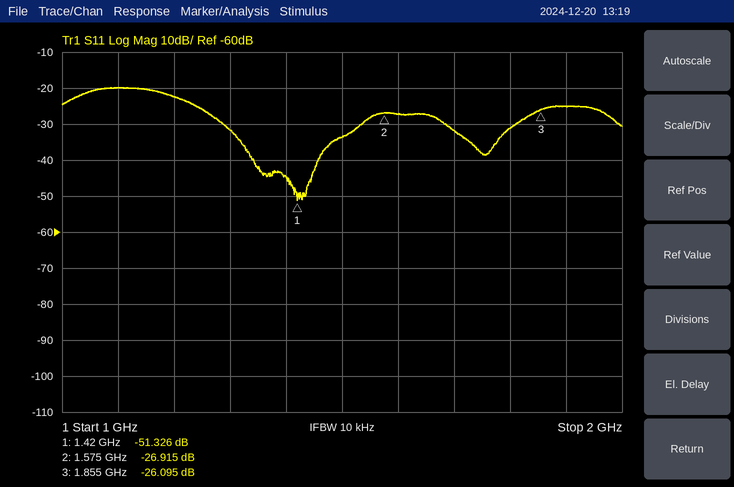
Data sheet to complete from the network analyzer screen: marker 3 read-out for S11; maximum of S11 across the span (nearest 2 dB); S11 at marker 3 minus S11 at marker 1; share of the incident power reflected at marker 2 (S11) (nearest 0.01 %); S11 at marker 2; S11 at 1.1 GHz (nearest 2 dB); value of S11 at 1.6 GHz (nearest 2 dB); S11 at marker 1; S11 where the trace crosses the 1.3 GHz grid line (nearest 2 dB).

-26.095 dB
-20 dB
25.231 dB
0.20 %
-26.915 dB
-20 dB
-28 dB
-51.326 dB
-32 dB
